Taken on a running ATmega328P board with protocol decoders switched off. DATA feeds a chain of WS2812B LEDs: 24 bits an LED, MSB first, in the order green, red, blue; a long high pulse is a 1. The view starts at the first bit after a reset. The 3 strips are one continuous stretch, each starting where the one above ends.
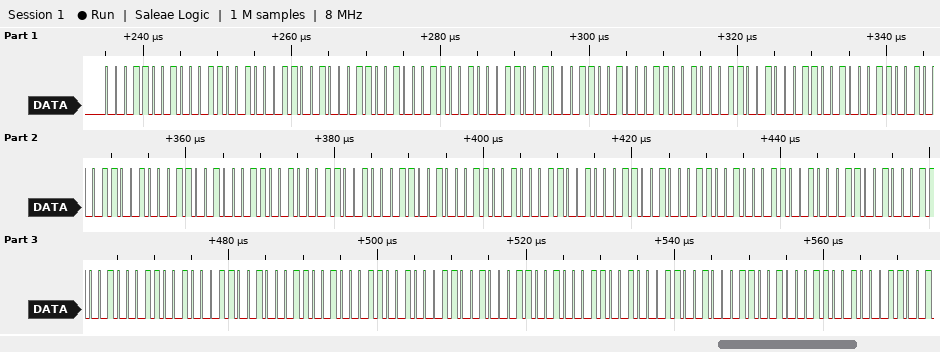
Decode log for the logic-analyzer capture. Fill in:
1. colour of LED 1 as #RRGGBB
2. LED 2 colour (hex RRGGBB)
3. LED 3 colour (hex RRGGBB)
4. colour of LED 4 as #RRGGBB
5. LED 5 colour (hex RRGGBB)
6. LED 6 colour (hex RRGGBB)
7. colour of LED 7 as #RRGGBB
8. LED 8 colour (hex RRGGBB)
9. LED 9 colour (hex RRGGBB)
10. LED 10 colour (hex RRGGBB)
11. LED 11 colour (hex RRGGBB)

#191919
#191919
#191919
#191919
#191919
#191919
#191919
#191919
#191919
#191919
#191919
